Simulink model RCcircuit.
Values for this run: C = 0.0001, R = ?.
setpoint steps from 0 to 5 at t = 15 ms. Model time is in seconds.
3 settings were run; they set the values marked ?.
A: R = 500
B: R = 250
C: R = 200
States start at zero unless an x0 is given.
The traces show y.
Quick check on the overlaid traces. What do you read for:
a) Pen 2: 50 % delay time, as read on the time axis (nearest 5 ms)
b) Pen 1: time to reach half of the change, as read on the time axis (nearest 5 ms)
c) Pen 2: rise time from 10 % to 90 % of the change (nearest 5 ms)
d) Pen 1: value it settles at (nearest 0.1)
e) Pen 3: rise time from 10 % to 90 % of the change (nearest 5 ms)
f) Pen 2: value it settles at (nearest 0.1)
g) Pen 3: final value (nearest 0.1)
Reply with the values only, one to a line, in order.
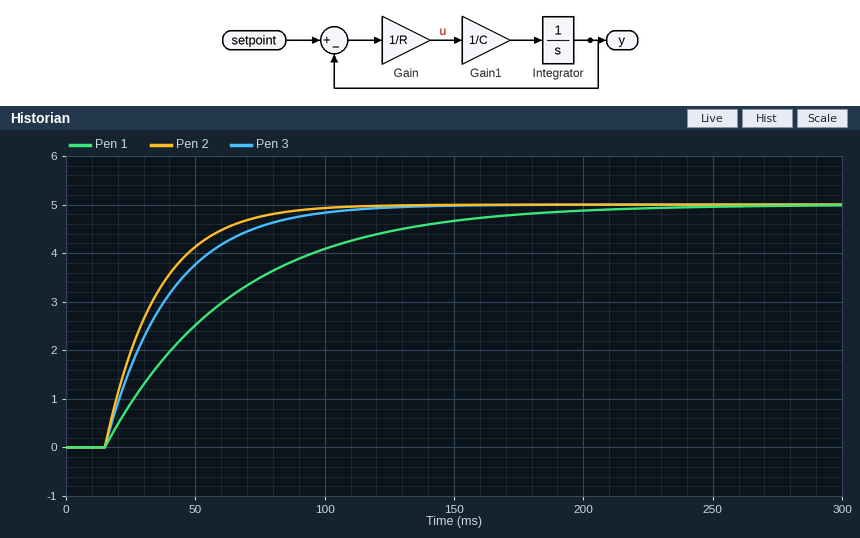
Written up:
30 ms
50 ms
45 ms
5.0
55 ms
5.0
5.0
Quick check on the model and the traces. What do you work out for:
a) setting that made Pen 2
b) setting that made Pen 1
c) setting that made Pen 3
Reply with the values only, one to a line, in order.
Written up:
C
A
B
